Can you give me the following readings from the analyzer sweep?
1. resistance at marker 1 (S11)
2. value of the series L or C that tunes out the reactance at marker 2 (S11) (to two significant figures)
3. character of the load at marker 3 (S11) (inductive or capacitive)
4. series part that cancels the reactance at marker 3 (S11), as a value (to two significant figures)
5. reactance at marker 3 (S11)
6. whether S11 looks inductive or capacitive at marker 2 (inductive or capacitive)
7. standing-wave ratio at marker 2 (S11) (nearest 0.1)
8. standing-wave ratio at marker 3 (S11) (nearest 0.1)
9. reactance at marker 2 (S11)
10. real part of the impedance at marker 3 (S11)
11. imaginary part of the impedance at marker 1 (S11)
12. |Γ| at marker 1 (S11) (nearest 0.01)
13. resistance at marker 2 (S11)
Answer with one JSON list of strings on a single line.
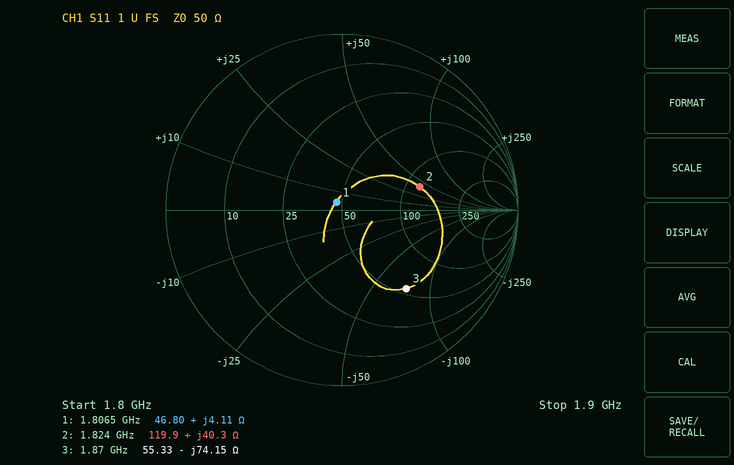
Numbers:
["46.80 Ω", "2.2 pF", "capacitive", "6.3 nH", "-74.15 Ω", "inductive", "2.7", "3.7", "+40.3 Ω", "55.33 Ω", "+4.11 Ω", "0.05", "119.9 Ω"]
